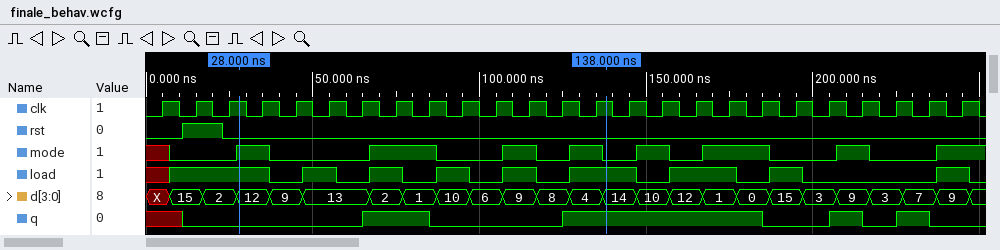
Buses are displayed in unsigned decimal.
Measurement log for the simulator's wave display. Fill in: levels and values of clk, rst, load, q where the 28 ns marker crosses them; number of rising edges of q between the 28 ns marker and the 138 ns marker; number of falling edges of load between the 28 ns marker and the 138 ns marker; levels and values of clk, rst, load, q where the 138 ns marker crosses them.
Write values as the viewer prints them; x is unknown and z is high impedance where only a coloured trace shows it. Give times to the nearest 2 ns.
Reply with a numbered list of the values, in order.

1. clk=1, rst=0, load=1, q=0
2. 2
3. 5
4. clk=1, rst=0, load=1, q=1
